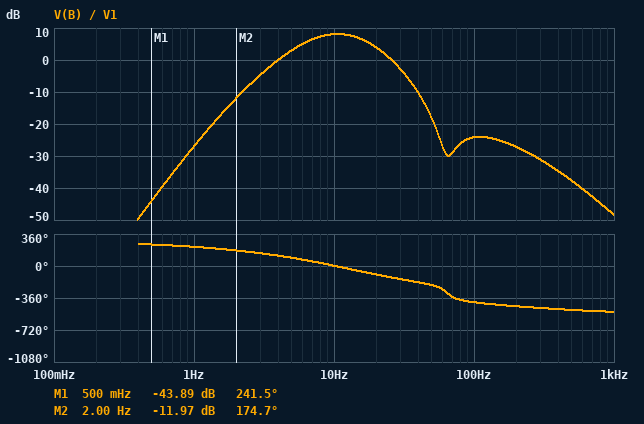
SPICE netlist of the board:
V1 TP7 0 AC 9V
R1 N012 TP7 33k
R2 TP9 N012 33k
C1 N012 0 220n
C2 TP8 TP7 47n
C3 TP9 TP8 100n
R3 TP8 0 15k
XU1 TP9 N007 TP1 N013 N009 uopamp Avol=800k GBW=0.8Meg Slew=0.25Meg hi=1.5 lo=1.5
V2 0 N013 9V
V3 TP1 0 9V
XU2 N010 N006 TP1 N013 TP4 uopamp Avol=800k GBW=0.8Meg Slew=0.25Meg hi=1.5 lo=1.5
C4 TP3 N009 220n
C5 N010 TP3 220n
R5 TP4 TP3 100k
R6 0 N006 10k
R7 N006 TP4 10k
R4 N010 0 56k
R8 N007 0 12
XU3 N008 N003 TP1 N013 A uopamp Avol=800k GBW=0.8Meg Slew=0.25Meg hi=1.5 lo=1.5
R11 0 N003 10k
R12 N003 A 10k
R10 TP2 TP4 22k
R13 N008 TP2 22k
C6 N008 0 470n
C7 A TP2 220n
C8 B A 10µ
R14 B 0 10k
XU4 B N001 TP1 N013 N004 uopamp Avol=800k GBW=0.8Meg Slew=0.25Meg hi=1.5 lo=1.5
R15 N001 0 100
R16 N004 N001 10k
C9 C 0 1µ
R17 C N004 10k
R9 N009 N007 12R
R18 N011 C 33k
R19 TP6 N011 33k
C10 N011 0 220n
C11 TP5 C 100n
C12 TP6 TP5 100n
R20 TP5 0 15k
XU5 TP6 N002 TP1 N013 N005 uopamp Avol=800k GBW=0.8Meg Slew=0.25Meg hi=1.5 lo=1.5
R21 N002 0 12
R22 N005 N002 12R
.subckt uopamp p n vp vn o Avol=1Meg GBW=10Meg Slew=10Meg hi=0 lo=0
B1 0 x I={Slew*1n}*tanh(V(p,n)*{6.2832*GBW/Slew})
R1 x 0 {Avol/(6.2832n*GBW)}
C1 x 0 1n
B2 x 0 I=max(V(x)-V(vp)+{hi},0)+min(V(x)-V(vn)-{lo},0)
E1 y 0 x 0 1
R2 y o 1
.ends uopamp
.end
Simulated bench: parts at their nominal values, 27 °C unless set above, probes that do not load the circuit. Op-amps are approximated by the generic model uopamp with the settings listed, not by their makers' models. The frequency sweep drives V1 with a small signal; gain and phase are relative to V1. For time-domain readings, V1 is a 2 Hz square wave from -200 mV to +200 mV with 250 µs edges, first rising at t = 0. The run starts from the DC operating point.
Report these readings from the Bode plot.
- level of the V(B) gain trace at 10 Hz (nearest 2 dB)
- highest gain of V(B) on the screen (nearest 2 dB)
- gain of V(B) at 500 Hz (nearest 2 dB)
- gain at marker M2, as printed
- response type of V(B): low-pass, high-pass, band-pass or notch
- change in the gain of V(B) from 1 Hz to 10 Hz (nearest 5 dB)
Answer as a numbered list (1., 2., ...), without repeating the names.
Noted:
1. 8 dB
2. 8 dB
3. -38 dB
4. -11.97 dB
5. band-pass
6. 35 dB
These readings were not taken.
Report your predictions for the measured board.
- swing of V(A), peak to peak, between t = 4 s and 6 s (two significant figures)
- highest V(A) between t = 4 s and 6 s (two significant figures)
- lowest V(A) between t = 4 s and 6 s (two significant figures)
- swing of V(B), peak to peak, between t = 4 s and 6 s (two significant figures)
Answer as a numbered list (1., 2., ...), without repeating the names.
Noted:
1. 1.0 V
2. 510 mV
3. -510 mV
4. 890 mV
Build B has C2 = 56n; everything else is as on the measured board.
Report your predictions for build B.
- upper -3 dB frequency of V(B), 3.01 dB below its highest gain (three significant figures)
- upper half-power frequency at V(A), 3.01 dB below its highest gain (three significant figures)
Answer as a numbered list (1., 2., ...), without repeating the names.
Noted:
1. 18.1 Hz
2. 18.0 Hz
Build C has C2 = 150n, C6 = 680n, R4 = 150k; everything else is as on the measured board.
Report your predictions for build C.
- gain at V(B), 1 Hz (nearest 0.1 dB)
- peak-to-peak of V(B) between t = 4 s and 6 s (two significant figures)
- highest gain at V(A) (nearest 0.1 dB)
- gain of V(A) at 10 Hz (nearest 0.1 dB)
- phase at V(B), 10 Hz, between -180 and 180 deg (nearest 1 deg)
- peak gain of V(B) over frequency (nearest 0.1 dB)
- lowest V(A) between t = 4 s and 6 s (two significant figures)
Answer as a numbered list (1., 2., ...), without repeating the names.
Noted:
1. -18.2 dB
2. 2.8 V
3. 22.6 dB
4. 13.8 dB
5. -79 deg
6. 22.3 dB
7. -1.5 V
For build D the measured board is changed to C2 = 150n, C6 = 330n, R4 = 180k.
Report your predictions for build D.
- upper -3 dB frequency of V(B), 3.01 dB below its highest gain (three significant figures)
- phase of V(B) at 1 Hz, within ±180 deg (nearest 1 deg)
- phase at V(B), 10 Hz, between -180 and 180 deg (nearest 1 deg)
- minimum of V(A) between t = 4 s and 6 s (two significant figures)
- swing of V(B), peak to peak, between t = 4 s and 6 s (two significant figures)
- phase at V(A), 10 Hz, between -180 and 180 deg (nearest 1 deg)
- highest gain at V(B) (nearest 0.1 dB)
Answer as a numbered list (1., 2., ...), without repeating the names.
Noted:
1. 5.87 Hz
2. -132 deg
3. -62 deg
4. -2.9 V
5. 5.7 V
6. -71 deg
7. 33.2 dB
